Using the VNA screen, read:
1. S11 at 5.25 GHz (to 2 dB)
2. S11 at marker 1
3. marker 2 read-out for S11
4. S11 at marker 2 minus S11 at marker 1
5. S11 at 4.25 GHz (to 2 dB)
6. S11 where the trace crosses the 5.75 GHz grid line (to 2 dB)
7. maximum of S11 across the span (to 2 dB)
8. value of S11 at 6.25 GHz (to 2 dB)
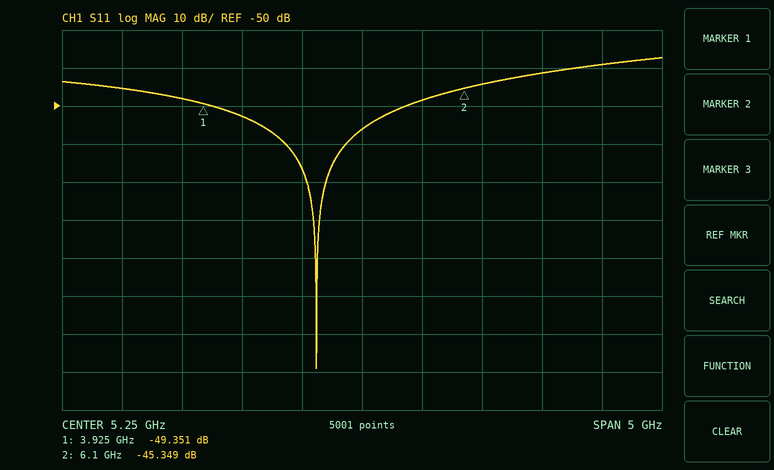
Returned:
-56 dB
-49.351 dB
-45.349 dB
4.002 dB
-52 dB
-48 dB
-38 dB
-44 dB
